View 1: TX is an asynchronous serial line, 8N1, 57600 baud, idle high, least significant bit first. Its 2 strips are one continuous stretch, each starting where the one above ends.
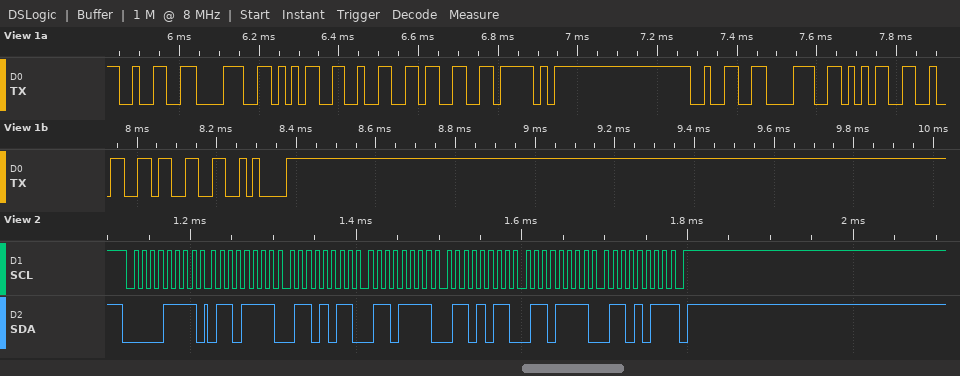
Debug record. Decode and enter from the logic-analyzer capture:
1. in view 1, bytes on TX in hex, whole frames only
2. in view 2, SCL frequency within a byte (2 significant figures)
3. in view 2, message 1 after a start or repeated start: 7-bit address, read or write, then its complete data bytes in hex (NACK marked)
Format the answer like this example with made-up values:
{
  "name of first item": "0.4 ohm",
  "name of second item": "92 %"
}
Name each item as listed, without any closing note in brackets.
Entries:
{
  "in view 1, bytes on TX in hex, whole frames only": "32 38 35 32 33 5F 32 38 35 32 33 0A",
  "in view 2, SCL frequency within a byte": "100 kHz",
  "in view 2, message 1 after a start or repeated start: 7-bit address, read or write, then its complete data bytes in hex": "0x07 read: 6F 6B 6F 6B 6F 6B NACK"
}
